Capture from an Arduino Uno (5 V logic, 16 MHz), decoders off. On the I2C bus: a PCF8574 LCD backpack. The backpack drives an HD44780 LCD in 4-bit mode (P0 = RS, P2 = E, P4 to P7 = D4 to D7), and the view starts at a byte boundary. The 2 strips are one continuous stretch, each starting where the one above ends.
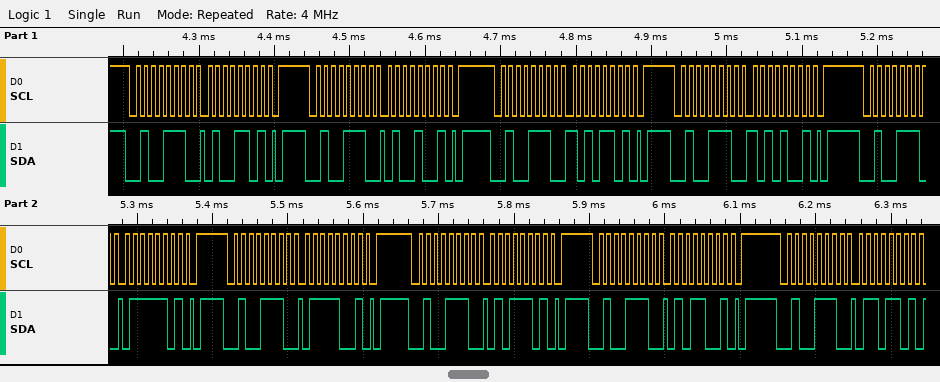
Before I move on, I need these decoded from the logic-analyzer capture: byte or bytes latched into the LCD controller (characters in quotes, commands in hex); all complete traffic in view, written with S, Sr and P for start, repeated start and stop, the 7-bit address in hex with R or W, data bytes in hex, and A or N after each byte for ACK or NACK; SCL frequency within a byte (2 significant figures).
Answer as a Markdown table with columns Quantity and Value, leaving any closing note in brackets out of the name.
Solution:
| Quantity | Value |
|---|---|
| byte or bytes latched into the LCD controller | 'J' 'u' |
| all complete traffic in view, written with S, Sr and P for start, repeated start and stop, the 7-bit address in hex with R or W, data bytes in hex, and A or N after each byte for ACK or NACK | S 27W A 4D A P S 27W A 49 A P S 27W A AD A P S 27W A A9 A P S 27W A 7D A P S 27W A 79 A P S 27W A 5D A P S 27W A 59 A P S 27W A 6D A |
| SCL frequency within a byte | 100 kHz |
